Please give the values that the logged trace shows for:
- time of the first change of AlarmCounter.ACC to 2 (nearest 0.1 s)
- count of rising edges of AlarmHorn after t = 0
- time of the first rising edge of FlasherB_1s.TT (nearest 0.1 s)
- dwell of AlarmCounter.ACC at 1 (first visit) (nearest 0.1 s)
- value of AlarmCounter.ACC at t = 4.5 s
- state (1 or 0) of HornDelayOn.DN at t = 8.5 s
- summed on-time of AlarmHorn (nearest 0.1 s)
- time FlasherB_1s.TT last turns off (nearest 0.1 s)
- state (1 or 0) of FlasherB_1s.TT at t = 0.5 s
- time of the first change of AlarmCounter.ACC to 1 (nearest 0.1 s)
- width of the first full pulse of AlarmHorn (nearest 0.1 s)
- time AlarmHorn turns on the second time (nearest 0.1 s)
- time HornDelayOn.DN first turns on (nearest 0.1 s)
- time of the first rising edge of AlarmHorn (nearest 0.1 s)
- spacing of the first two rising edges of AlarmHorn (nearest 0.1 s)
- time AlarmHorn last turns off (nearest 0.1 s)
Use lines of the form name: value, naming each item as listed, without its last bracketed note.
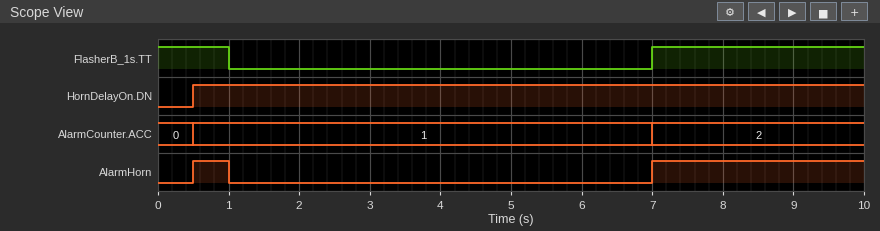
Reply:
time of the first change of AlarmCounter.ACC to 2: 7.0 s
count of rising edges of AlarmHorn after t = 0: 2
time of the first rising edge of FlasherB_1s.TT: 7.0 s
dwell of AlarmCounter.ACC at 1 (first visit): 6.5 s
value of AlarmCounter.ACC at t = 4.5 s: 1
state (1 or 0) of HornDelayOn.DN at t = 8.5 s: 1
summed on-time of AlarmHorn: 3.5 s
time FlasherB_1s.TT last turns off: 1.0 s
state (1 or 0) of FlasherB_1s.TT at t = 0.5 s: 1
time of the first change of AlarmCounter.ACC to 1: 0.5 s
width of the first full pulse of AlarmHorn: 0.5 s
time AlarmHorn turns on the second time: 7.0 s
time HornDelayOn.DN first turns on: 0.5 s
time of the first rising edge of AlarmHorn: 0.5 s
spacing of the first two rising edges of AlarmHorn: 6.5 s
time AlarmHorn last turns off: 1.0 s
